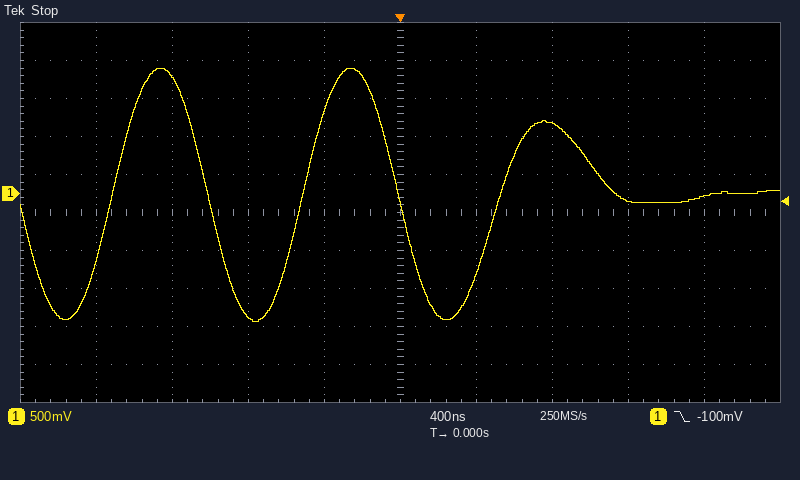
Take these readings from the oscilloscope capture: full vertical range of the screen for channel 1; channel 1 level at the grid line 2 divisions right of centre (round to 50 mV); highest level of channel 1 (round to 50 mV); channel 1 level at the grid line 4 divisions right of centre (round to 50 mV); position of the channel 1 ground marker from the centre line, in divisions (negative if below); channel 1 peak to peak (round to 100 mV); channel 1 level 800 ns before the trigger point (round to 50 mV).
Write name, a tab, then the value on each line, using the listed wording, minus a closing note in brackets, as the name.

full vertical range of the screen for channel 1	5 V
channel 1 level at the grid line 2 divisions right of centre	900 mV
highest level of channel 1	1.65 V
channel 1 level at the grid line 4 divisions right of centre	-50 mV
position of the channel 1 ground marker from the centre line, in divisions	+0.5 div
channel 1 peak to peak	3.30 V
channel 1 level 800 ns before the trigger point	-1.60 V
